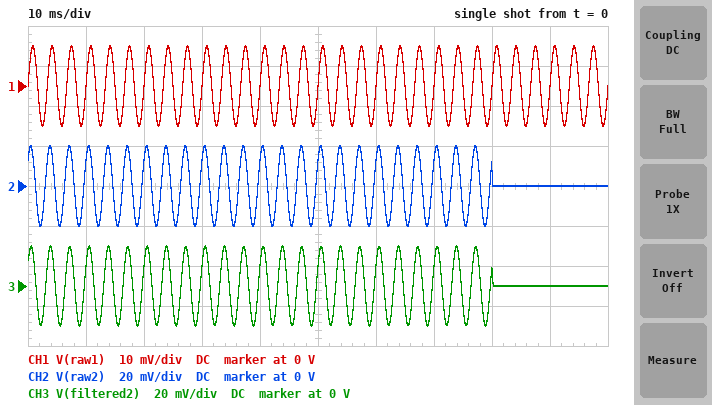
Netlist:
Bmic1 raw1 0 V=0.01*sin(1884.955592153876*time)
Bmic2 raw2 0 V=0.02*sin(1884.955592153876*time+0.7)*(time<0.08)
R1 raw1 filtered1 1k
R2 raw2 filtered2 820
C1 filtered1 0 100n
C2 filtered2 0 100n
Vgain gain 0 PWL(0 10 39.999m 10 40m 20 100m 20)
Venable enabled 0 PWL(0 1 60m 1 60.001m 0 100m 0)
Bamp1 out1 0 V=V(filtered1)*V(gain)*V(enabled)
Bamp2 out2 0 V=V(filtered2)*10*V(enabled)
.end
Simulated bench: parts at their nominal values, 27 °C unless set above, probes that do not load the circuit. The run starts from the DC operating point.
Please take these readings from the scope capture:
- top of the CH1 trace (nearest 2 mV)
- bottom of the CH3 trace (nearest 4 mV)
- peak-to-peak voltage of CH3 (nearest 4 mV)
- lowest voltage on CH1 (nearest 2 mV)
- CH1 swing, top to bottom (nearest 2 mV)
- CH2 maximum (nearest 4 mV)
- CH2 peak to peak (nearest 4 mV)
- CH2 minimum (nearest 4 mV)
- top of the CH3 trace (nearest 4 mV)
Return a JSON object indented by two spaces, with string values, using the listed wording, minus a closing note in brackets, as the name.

{
  "top of the CH1 trace": "10 mV",
  "bottom of the CH3 trace": "-20 mV",
  "peak-to-peak voltage of CH3": "40 mV",
  "lowest voltage on CH1": "-10 mV",
  "CH1 swing, top to bottom": "20 mV",
  "CH2 maximum": "20 mV",
  "CH2 peak to peak": "40 mV",
  "CH2 minimum": "-20 mV",
  "top of the CH3 trace": "20 mV"
}
